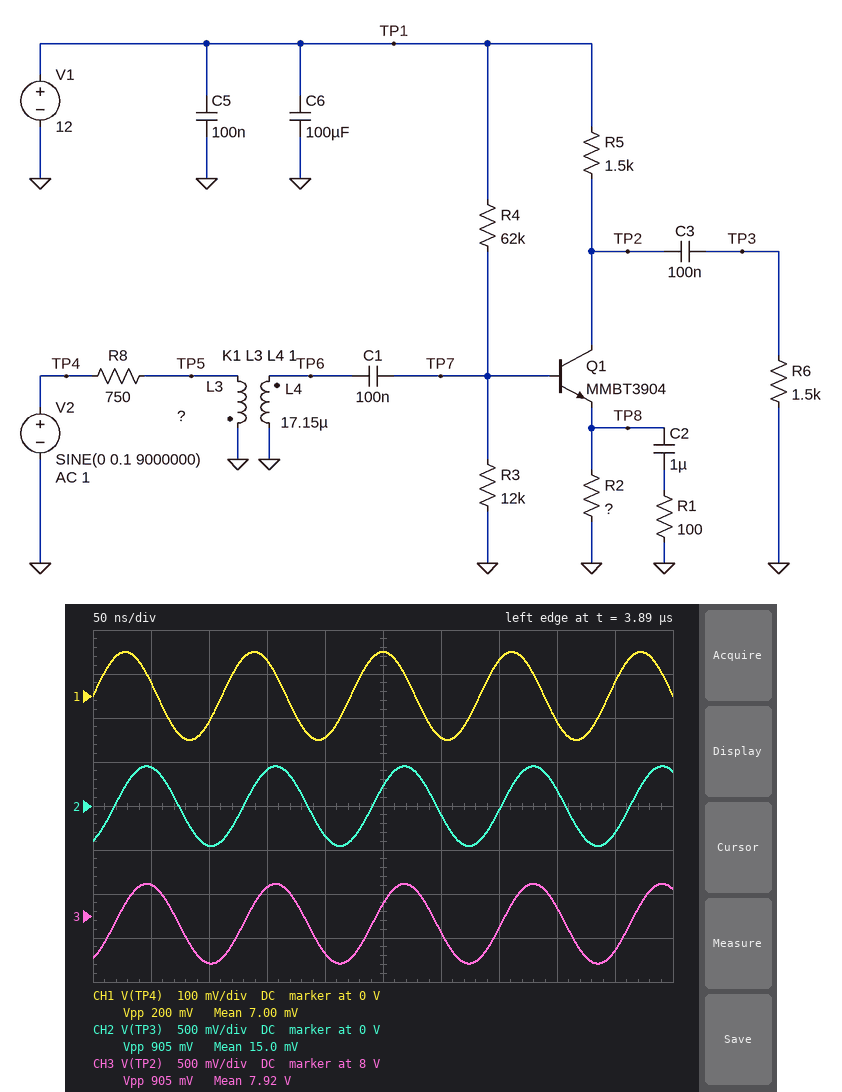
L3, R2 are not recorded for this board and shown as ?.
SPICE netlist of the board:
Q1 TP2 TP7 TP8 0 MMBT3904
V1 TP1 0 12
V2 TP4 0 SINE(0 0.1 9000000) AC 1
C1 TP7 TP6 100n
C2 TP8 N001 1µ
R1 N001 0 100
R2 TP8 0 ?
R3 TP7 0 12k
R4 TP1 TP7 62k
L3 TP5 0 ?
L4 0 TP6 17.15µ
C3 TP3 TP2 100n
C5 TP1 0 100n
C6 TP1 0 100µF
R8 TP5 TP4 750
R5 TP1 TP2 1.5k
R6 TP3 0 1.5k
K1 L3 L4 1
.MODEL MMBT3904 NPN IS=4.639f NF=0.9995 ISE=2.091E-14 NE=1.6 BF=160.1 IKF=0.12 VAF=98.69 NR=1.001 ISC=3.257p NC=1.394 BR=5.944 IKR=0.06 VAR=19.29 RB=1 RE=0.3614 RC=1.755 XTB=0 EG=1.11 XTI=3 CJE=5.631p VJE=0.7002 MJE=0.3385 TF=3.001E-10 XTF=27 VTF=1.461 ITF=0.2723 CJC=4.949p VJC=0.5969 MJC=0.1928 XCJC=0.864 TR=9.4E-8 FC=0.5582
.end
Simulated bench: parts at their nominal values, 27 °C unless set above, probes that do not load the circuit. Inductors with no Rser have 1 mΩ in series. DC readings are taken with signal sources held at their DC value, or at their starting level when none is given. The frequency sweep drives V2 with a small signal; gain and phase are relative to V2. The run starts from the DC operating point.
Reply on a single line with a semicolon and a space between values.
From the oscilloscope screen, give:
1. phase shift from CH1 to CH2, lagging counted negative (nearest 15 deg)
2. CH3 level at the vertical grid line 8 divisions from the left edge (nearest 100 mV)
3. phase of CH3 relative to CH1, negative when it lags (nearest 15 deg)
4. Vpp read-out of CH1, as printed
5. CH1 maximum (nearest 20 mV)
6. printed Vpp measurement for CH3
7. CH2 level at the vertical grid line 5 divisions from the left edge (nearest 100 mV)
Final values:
-60 deg; 8.1 V; -60 deg; 200 mV; 100 mV; 905 mV; 200 mV
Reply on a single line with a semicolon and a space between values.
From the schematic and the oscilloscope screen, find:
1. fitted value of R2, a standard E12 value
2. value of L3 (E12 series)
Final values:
390 Ω; 3.3 µH
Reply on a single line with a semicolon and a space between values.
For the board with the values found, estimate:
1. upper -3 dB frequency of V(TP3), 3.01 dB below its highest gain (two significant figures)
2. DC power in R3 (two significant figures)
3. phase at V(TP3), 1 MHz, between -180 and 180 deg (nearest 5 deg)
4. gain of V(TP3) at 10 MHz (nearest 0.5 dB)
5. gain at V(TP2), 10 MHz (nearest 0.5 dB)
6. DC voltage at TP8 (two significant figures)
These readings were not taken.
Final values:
8.0 MHz; 260 µW; 85 deg; 11.0 dB; 11.0 dB; 1.1 V
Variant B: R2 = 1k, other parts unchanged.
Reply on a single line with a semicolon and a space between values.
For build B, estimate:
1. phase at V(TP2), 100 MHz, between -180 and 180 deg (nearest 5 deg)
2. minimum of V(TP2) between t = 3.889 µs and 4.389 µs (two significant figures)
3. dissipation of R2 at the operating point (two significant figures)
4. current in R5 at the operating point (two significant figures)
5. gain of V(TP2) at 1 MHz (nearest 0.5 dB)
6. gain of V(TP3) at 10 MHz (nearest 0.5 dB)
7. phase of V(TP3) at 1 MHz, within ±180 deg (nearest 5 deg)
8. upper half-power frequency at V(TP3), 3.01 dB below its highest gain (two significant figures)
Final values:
-115 deg; 9.7 V; 1.4 mW; 1.2 mA; -7.5 dB; 12.0 dB; 85 deg; 9.0 MHz
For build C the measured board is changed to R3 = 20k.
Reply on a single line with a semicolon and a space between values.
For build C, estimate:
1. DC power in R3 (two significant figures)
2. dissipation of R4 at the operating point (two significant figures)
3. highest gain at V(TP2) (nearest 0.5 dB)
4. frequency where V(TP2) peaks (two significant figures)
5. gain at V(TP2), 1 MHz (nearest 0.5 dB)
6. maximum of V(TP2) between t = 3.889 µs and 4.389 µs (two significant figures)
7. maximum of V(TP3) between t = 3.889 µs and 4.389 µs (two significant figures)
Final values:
310 µW; 1.5 mW; 19.0 dB; 6.1 MHz; -5.0 dB; 5.7 V; 380 mV
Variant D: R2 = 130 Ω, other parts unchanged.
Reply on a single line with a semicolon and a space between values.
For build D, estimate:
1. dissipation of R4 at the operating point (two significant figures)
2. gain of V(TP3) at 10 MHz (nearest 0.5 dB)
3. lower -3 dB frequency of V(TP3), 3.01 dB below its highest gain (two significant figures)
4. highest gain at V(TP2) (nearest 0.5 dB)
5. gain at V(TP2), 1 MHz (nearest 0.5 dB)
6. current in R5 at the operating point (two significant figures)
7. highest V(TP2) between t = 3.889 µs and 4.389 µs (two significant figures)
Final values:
1.8 mW; 8.0 dB; 4.2 MHz; 20.5 dB; -2.0 dB; 6.1 mA; 3.1 V
